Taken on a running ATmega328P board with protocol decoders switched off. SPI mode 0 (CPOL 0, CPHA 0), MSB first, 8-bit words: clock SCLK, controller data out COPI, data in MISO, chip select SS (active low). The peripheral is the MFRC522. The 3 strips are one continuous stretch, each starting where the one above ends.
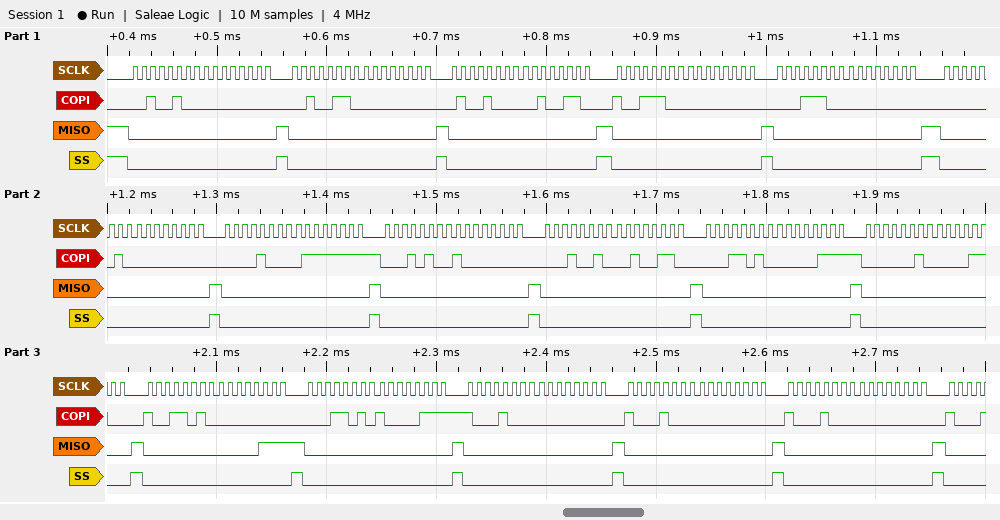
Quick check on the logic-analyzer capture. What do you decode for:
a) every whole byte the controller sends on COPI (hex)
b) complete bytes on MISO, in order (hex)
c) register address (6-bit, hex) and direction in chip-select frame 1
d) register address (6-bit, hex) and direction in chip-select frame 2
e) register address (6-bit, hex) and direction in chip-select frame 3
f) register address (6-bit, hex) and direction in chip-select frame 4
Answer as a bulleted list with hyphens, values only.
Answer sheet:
- 24 00 26 00 48 26 9C 00 1C 00 02 00 08 7F 14 80 12 26 1A 07 02 0C 9A 00 1A 87 88 00 88 00 88 00
- 00 00 00 00 00 00 00 00 00 00 00 00 00 00 00 00 00 00 00 00 00 00 00 07 00 00 00 00 00 00 00 00
- 0x12 write
- 0x13 write
- 0x24 write
- 0x0E read
